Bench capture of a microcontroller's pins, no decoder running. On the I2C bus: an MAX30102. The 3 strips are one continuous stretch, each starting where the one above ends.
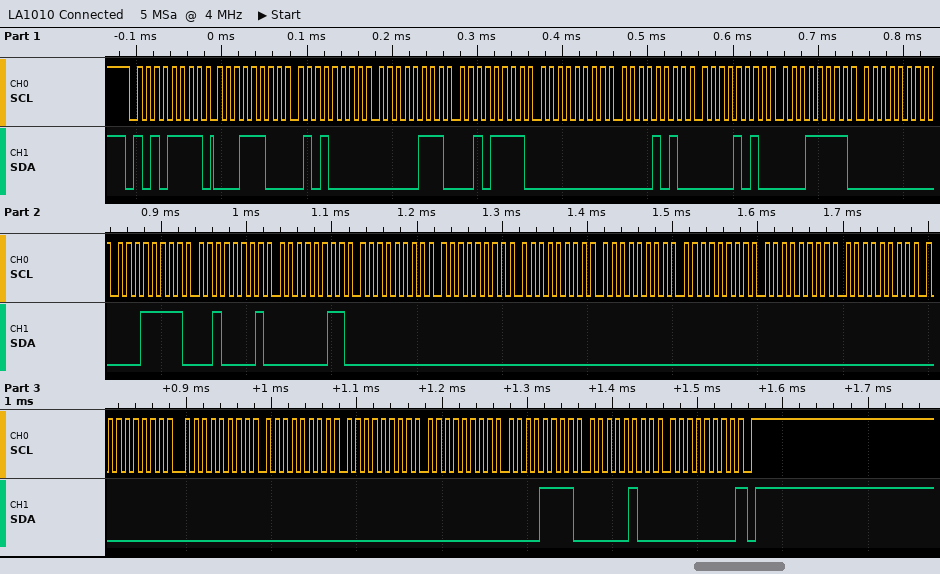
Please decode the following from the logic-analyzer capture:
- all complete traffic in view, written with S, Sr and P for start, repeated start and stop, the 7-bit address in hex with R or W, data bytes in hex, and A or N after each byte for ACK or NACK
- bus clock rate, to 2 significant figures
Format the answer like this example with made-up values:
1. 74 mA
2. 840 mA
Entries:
1. S 57R A 1C A 50 A 07 A 2F A 00 A 0A A 0A A 1F A 00 A 1F A 21 A 03 A 00 A 00 A 00 A 00 A 00 A 00 A 00 A 00 A 00 A 00 A 00 A 00 A 0F A 04 A 00 N P
2. 100 kHz
